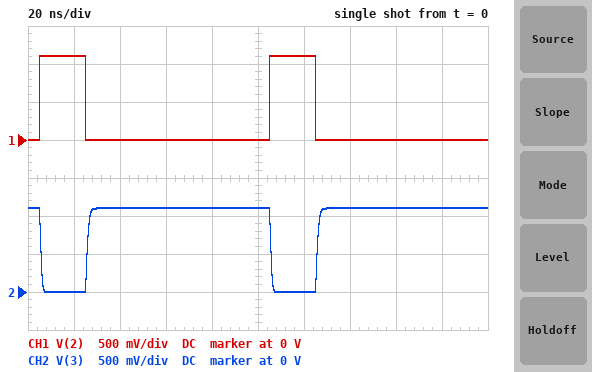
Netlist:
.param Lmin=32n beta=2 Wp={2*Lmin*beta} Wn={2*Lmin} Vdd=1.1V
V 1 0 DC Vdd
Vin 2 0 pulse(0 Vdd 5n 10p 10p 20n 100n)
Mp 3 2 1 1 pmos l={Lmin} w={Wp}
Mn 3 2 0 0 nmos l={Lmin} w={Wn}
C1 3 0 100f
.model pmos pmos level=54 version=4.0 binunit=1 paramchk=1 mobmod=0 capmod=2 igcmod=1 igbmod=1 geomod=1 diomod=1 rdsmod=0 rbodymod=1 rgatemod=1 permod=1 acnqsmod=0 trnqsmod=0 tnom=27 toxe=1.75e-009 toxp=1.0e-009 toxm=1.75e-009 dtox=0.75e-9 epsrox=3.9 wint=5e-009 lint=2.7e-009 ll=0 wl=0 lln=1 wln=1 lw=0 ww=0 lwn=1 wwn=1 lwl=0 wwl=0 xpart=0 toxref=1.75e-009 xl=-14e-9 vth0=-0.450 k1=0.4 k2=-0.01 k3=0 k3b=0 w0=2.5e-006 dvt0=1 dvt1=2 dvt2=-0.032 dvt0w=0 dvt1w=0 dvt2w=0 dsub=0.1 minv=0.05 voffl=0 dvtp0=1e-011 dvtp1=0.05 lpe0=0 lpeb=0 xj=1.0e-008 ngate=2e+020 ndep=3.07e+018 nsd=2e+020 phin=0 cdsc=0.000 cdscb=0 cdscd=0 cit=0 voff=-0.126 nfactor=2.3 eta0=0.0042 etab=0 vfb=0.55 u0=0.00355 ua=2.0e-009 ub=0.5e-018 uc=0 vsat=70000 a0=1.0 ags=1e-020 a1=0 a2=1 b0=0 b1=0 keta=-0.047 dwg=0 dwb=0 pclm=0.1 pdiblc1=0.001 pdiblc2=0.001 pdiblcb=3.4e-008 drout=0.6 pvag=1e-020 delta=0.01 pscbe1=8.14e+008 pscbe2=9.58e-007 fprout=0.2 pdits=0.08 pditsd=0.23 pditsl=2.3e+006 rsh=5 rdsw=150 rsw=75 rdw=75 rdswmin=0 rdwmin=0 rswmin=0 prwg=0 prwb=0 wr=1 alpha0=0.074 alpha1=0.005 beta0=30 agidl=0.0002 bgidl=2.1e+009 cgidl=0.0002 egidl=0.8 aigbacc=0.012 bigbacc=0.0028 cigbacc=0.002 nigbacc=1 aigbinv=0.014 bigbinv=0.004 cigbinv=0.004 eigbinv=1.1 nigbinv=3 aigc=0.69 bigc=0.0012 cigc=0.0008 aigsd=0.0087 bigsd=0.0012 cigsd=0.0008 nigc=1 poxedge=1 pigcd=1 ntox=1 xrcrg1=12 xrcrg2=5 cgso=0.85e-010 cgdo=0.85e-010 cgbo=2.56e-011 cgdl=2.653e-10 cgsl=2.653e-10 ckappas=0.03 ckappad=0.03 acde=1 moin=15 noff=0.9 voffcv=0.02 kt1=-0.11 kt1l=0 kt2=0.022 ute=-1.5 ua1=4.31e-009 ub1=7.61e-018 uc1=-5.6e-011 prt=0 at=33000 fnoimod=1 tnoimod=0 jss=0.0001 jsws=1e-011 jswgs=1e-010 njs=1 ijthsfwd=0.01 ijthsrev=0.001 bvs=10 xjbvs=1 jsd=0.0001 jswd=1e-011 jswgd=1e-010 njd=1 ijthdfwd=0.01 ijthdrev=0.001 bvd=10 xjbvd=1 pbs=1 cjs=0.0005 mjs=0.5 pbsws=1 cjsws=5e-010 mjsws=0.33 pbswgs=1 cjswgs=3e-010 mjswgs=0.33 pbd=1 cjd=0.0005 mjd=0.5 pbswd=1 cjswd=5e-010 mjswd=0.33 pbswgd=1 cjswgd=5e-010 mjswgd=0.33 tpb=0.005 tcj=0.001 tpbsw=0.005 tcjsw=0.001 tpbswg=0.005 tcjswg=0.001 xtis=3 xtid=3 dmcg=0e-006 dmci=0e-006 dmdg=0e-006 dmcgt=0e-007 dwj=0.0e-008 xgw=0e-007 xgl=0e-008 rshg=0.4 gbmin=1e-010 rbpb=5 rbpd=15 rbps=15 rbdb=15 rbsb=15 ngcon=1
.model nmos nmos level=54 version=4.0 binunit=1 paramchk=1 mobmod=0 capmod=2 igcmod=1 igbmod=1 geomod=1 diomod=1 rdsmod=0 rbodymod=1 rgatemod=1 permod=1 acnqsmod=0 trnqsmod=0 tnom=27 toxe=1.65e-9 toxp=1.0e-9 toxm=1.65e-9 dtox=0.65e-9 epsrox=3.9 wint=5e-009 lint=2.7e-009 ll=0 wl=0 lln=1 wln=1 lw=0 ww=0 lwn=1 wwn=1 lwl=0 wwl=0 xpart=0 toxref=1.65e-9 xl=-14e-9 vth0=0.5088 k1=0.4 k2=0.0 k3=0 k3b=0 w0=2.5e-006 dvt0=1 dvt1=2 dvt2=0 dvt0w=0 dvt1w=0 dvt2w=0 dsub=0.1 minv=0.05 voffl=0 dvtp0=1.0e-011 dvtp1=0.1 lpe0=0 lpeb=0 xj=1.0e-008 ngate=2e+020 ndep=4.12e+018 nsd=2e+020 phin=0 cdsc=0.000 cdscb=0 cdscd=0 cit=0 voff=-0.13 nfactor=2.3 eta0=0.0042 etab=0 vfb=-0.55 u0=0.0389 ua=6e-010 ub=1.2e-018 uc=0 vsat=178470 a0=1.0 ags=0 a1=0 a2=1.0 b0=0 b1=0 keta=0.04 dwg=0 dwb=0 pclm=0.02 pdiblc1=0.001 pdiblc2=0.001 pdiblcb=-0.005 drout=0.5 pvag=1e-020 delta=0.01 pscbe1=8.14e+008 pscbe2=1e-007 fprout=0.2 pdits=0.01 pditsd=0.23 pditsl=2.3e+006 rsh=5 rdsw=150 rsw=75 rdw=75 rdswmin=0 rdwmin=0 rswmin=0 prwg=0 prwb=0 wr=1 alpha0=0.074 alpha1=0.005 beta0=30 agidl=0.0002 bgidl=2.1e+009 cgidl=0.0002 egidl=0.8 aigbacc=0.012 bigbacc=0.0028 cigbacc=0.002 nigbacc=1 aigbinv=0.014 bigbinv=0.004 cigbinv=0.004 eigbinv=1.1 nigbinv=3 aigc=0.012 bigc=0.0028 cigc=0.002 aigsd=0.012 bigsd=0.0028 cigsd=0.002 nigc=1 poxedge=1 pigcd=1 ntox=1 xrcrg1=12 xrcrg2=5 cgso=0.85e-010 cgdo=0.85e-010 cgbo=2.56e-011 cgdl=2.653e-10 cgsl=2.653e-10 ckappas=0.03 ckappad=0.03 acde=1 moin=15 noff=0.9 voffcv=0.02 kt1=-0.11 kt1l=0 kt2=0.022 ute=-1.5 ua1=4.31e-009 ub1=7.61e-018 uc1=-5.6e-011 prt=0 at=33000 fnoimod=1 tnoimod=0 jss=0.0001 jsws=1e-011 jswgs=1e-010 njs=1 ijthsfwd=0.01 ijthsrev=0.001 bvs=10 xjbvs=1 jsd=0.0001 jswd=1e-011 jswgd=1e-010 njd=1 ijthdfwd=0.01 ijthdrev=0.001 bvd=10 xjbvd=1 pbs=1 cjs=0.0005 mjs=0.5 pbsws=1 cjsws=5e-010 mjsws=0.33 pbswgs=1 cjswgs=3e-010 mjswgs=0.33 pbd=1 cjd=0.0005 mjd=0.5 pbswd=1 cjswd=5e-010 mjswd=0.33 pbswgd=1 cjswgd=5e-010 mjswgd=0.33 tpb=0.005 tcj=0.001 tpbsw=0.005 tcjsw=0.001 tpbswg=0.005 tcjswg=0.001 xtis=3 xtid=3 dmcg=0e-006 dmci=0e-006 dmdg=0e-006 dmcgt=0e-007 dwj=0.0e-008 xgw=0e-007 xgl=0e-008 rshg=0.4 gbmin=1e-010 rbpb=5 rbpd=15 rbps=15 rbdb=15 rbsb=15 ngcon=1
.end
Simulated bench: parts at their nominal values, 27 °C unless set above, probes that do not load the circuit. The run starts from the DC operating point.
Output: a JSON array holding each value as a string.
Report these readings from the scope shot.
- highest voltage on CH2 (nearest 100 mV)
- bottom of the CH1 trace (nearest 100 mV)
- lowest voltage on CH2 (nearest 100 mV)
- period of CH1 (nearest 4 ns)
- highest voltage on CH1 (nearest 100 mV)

["1.1 V", "0 V", "0 V", "100 ns", "1.1 V"]
